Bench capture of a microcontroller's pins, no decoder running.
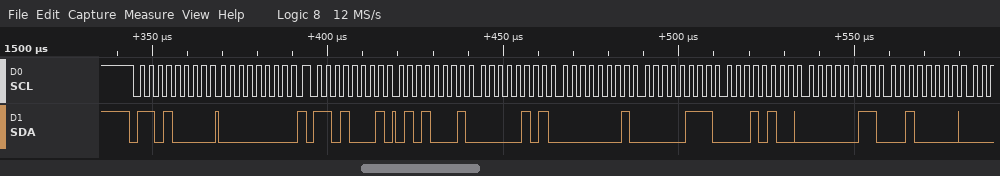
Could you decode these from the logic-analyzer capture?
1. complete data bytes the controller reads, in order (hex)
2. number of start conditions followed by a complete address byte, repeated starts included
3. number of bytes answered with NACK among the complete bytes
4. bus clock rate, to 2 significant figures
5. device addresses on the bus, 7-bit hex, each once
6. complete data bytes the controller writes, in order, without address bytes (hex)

51 05 01 07 14 03 20
2
0
400 kHz
0x68
00
